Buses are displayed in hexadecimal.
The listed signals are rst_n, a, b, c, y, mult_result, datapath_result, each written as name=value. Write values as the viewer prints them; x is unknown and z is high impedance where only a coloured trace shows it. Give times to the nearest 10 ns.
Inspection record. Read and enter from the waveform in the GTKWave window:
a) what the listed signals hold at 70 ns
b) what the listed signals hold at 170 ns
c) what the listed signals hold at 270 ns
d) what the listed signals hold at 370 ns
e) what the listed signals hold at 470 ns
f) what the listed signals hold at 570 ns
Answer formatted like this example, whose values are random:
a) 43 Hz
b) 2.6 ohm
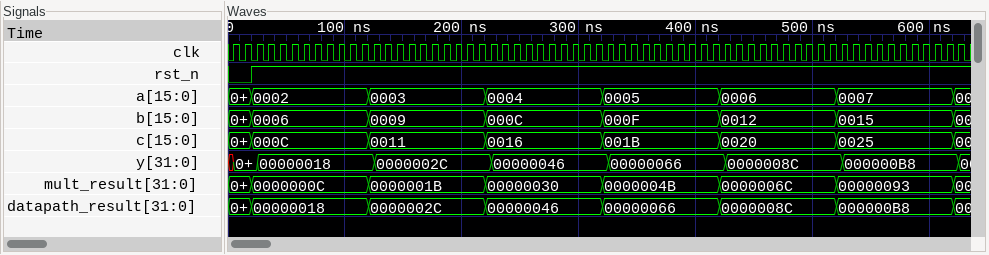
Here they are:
a) rst_n=1, a=0002, b=0006, c=000C, y=00000018, mult_result=0000000C, datapath_result=00000018
b) rst_n=1, a=0003, b=0009, c=0011, y=0000002C, mult_result=0000001B, datapath_result=0000002C
c) rst_n=1, a=0004, b=000C, c=0016, y=00000046, mult_result=00000030, datapath_result=00000046
d) rst_n=1, a=0005, b=000F, c=001B, y=00000066, mult_result=0000004B, datapath_result=00000066
e) rst_n=1, a=0006, b=0012, c=0020, y=0000008C, mult_result=0000006C, datapath_result=0000008C
f) rst_n=1, a=0007, b=0015, c=0025, y=000000B8, mult_result=00000093, datapath_result=000000B8
